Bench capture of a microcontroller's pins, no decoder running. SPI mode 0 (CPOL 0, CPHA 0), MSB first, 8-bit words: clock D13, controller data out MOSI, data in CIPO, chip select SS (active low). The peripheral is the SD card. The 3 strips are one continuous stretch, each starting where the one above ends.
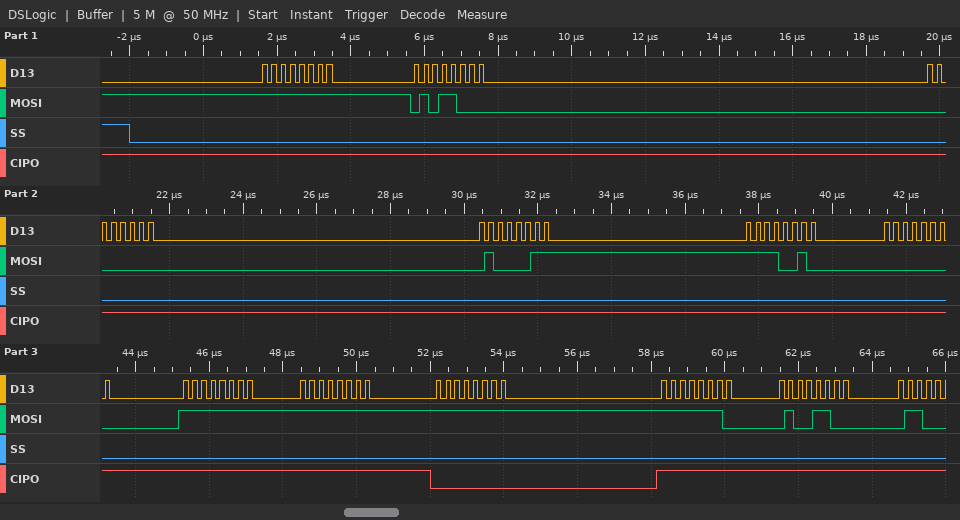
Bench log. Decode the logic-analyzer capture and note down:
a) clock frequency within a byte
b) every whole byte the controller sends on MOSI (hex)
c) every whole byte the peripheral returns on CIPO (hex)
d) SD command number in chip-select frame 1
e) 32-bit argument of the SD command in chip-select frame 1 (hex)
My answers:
4 MHz
0xFF 0x58 0x00 0x43 0xF2 0x00 0xFF 0xFF 0xFF 0xFE 0x4C
0xFF 0xFF 0xFF 0xFF 0xFF 0xFF 0xFF 0xFF 0x00 0xFF 0xFF
CMD24
0x0043F200
